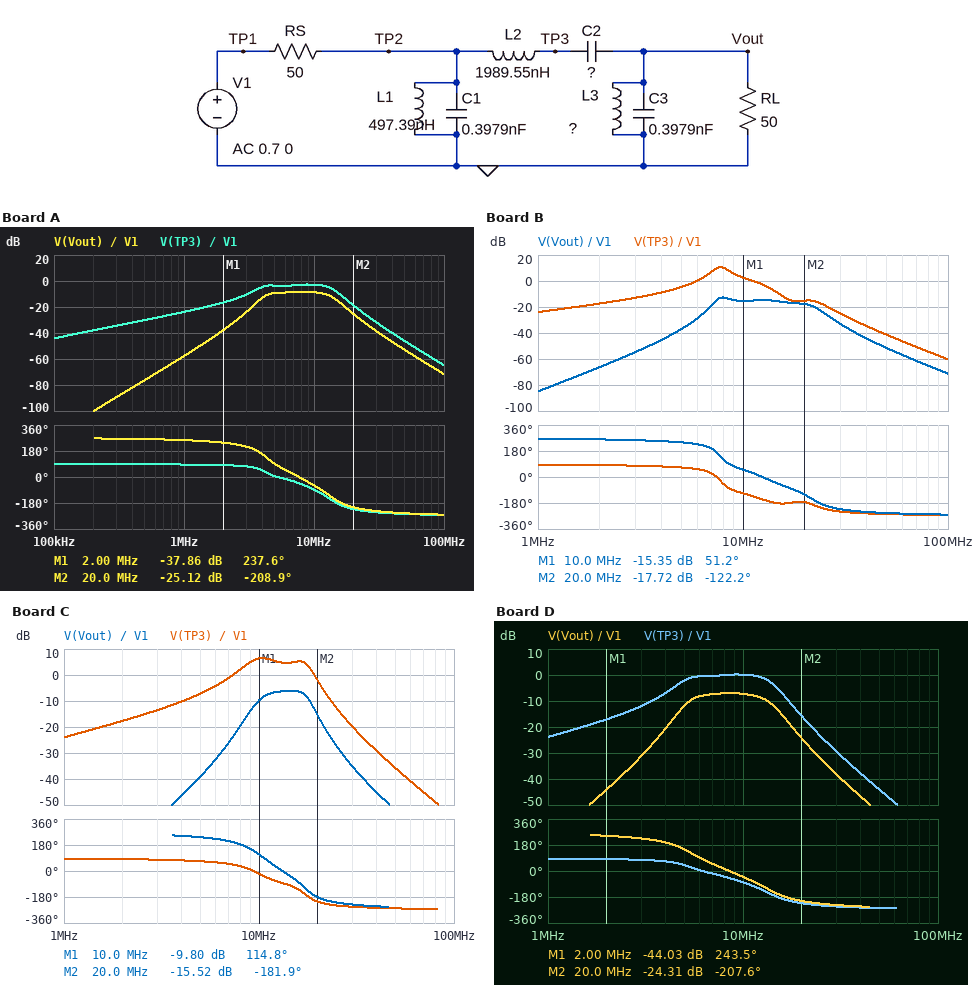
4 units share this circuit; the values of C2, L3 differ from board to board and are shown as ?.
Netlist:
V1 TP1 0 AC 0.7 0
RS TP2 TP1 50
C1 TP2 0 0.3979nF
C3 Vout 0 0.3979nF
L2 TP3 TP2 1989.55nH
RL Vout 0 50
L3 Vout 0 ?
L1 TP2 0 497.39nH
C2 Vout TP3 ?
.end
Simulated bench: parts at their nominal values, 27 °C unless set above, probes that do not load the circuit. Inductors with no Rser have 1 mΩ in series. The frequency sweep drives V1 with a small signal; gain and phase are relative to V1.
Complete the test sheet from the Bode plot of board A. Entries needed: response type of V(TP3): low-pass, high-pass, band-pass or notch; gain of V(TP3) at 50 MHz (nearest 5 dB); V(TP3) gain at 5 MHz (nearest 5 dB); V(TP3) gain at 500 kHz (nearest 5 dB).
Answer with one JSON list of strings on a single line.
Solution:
["band-pass", "-45 dB", "-5 dB", "-30 dB"]
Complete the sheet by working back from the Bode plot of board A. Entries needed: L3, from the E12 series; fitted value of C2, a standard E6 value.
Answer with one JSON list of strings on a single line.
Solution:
["1.5 µH", "330 pF"]
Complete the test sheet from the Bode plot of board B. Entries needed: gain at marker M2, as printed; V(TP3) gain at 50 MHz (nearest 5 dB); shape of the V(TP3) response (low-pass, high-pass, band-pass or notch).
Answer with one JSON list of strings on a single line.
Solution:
["-17.72 dB", "-40 dB", "band-pass"]
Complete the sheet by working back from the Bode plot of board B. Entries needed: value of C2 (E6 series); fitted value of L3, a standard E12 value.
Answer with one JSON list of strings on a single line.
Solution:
["150 pF", "150 nH"]
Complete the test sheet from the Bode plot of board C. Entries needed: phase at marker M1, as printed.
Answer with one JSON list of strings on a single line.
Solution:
["114.8 deg"]
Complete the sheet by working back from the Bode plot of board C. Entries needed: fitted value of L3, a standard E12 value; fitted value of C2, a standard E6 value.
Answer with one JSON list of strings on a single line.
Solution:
["330 nH", "68 pF"]
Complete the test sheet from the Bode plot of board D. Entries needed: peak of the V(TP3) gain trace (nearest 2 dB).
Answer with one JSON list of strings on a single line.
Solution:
["0 dB"]
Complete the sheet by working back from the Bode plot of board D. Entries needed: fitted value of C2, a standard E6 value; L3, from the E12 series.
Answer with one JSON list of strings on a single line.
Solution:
["220 pF", "1.2 µH"]
